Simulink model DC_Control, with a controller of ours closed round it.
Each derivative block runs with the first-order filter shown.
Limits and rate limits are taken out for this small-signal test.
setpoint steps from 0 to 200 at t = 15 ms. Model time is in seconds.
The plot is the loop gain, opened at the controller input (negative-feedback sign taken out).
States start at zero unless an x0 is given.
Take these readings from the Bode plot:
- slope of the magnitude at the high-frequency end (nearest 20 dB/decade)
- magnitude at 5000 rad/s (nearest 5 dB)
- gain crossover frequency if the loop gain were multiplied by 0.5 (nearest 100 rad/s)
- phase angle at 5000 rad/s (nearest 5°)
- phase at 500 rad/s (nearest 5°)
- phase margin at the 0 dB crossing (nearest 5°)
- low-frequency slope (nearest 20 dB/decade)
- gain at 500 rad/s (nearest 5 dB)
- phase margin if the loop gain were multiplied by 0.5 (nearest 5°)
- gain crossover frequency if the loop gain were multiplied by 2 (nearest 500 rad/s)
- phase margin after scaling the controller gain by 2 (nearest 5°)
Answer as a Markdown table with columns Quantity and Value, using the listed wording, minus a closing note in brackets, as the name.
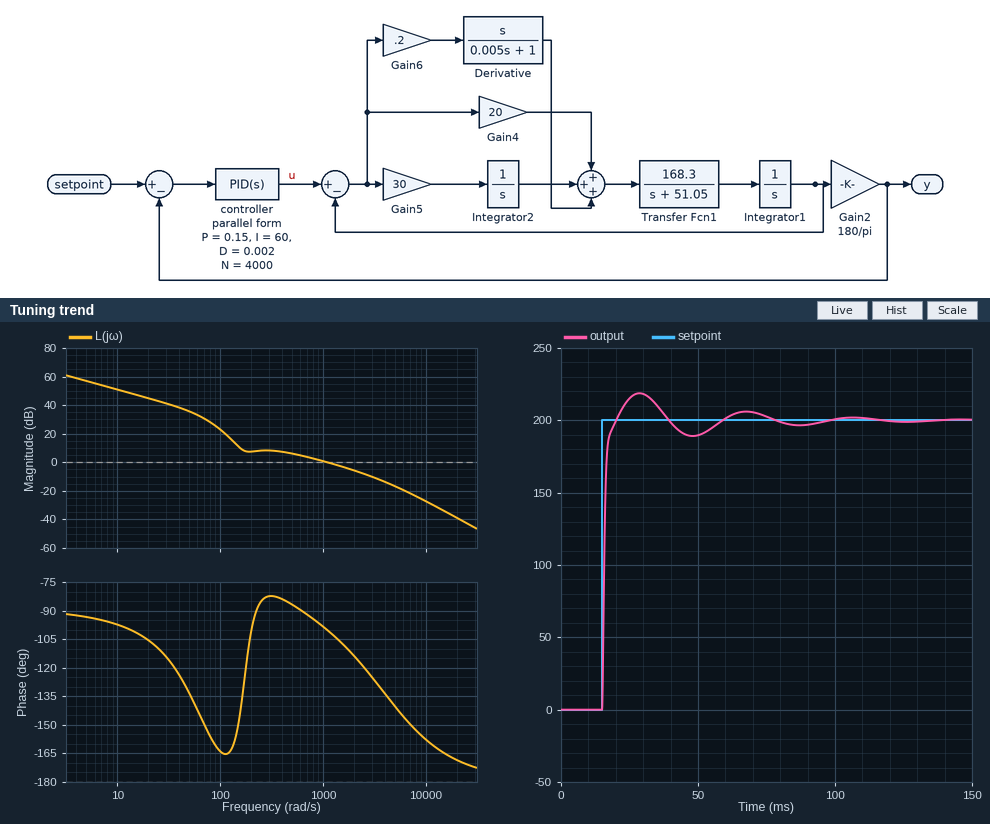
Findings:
| Quantity | Value |
|---|---|
| slope of the magnitude at the high-frequency end | -40 dB/decade |
| magnitude at 5000 rad/s | -15 dB |
| gain crossover frequency if the loop gain were multiplied by 0.5 | 500 rad/s |
| phase angle at 5000 rad/s | -140° |
| phase at 500 rad/s | -85° |
| phase margin at the 0 dB crossing | 80° |
| low-frequency slope | -20 dB/decade |
| gain at 500 rad/s | 5 dB |
| phase margin if the loop gain were multiplied by 0.5 | 95° |
| gain crossover frequency if the loop gain were multiplied by 2 | 2000 rad/s |
| phase margin after scaling the controller gain by 2 | 65° |
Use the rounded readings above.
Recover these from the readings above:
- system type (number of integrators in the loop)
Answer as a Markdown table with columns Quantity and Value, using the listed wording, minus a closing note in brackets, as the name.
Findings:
| Quantity | Value |
|---|---|
| system type | 1 |
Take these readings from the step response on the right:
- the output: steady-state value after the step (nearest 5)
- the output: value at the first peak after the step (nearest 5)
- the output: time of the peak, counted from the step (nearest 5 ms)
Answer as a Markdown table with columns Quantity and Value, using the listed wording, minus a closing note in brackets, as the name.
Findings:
| Quantity | Value |
|---|---|
| the output: steady-state value after the step | 200 |
| the output: value at the first peak after the step | 220 |
| the output: time of the peak, counted from the step | 15 ms |
